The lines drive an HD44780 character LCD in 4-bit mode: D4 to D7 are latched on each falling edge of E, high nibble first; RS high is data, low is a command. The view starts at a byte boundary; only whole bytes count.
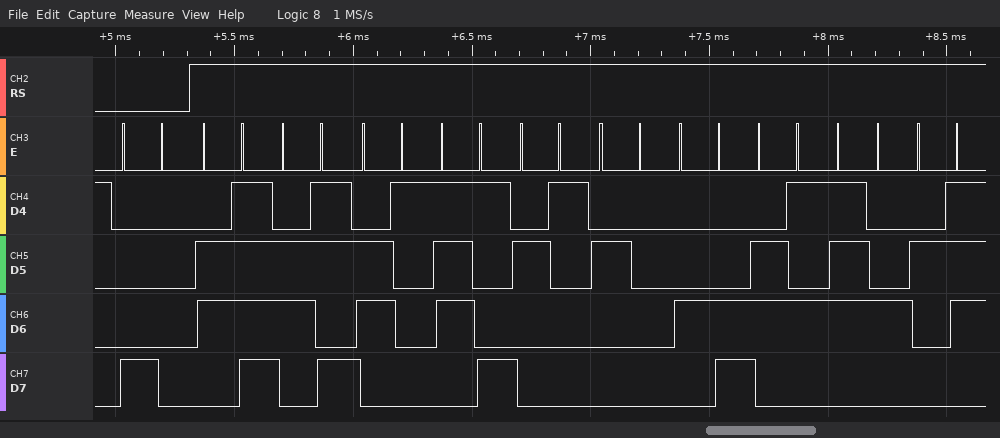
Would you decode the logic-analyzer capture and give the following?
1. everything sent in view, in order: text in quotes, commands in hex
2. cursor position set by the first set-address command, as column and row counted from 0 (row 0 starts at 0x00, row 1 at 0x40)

0x80 "okay! Let'"
column 0, row 0
